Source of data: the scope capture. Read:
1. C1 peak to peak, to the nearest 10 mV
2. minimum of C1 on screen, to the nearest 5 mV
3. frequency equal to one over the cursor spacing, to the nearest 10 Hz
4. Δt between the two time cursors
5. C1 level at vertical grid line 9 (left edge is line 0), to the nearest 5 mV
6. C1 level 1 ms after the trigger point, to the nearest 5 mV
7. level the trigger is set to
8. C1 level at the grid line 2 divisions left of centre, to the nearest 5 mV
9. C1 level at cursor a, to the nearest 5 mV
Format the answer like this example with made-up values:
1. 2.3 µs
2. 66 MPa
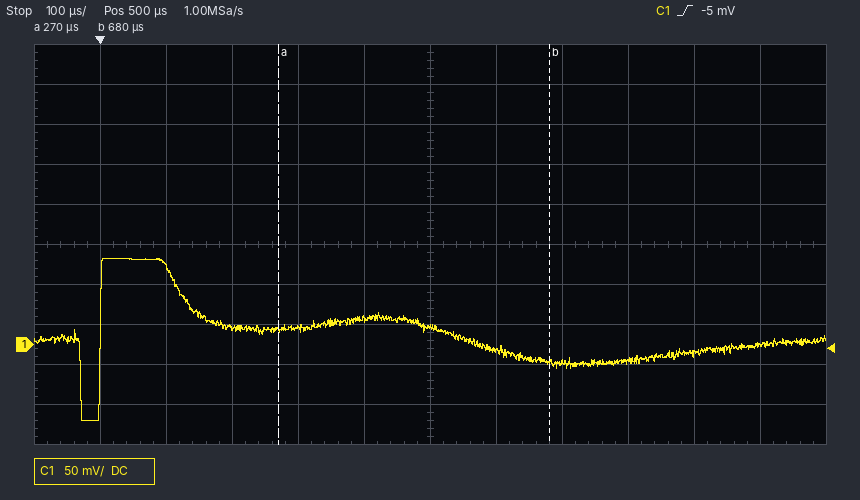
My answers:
1. 200 mV
2. -95 mV
3. 2.44 kHz
4. 410 µs
5. -20 mV
6. 0 mV
7. -5 mV
8. 20 mV
9. 20 mV
